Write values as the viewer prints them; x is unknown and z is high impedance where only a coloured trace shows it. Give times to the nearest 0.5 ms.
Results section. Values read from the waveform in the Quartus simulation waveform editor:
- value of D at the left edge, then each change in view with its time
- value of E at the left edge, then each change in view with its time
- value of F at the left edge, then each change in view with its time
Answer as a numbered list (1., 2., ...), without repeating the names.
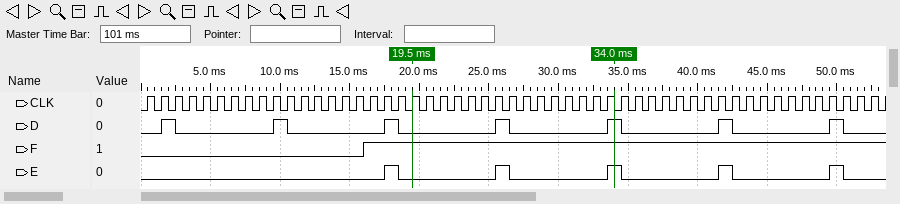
1. 0, 1 at 1.5 ms, 0 at 2.5 ms, 1 at 9.5 ms, 0 at 10.5 ms, 1 at 17.5 ms, 0 at 18.5 ms, 1 at 25.5 ms, 0 at 26.5 ms, 1 at 33.5 ms, 0 at 34.5 ms, 1 at 41.5 ms, 0 at 42.5 ms, 1 at 49.5 ms, 0 at 50.5 ms
2. 0, 1 at 17.5 ms, 0 at 18.5 ms, 1 at 25.5 ms, 0 at 26.5 ms, 1 at 33.5 ms, 0 at 34.5 ms, 1 at 41.5 ms, 0 at 42.5 ms, 1 at 49.5 ms, 0 at 50.5 ms
3. 0, 1 at 16 ms
